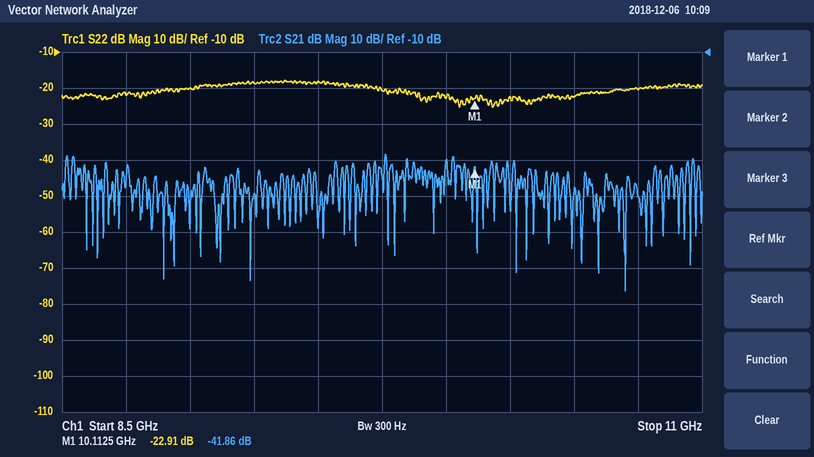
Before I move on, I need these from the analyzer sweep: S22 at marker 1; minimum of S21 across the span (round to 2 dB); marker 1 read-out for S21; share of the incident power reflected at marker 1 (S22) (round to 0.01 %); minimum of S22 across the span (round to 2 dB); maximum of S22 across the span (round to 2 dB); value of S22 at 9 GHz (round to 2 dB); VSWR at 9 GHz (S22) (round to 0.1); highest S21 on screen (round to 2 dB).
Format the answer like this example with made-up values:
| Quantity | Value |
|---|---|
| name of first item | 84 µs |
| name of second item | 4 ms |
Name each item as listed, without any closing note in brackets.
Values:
| Quantity | Value |
|---|---|
| S22 at marker 1 | -22.91 dB |
| minimum of S21 across the span | -76 dB |
| marker 1 read-out for S21 | -41.86 dB |
| share of the incident power reflected at marker 1 (S22) | 0.51 % |
| minimum of S22 across the span | -26 dB |
| maximum of S22 across the span | -18 dB |
| value of S22 at 9 GHz | -20 dB |
| VSWR at 9 GHz (S22) | 1.2 |
| highest S21 on screen | -38 dB |
